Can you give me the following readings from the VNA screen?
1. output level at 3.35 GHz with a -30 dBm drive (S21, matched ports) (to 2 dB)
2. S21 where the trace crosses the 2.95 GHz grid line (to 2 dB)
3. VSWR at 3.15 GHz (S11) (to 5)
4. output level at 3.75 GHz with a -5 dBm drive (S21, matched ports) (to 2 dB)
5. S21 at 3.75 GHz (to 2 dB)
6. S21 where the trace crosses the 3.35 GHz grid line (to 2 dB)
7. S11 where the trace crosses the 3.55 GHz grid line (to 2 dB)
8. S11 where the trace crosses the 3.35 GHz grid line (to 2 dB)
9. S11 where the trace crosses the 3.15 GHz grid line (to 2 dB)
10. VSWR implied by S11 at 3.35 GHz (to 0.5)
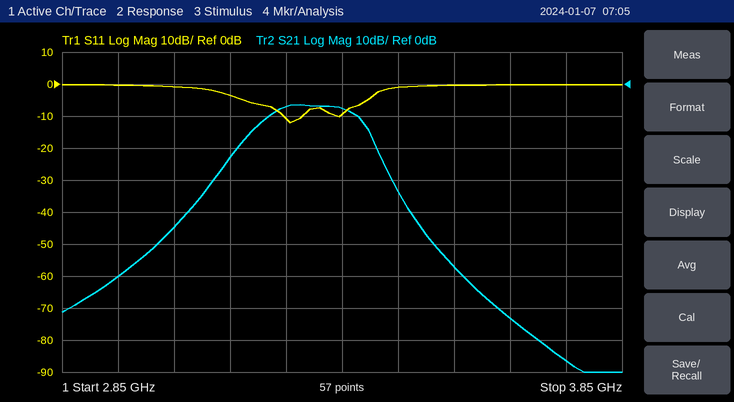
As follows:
-38 dBm
-60 dB
5
-92 dBm
-86 dB
-8 dB
0 dB
-10 dB
-4 dB
2.0
